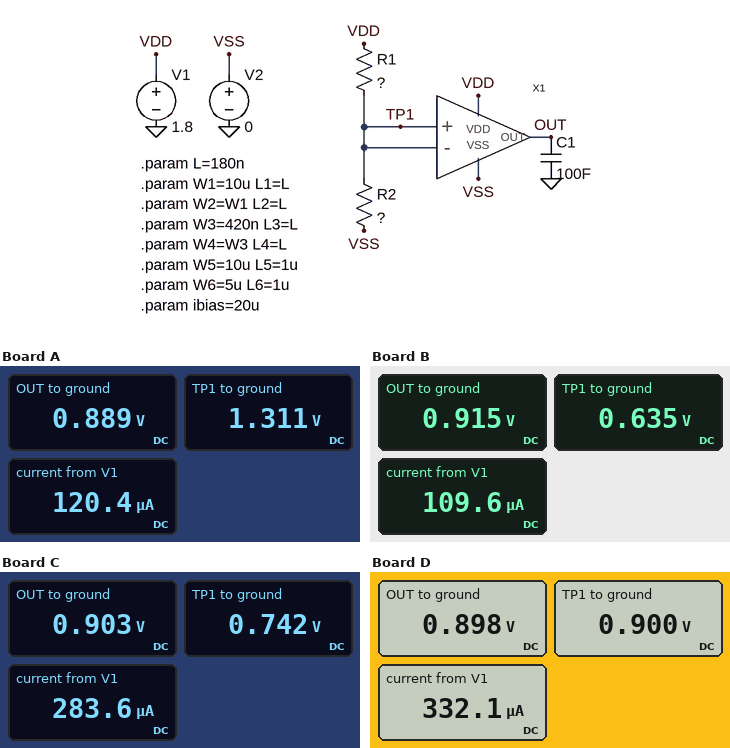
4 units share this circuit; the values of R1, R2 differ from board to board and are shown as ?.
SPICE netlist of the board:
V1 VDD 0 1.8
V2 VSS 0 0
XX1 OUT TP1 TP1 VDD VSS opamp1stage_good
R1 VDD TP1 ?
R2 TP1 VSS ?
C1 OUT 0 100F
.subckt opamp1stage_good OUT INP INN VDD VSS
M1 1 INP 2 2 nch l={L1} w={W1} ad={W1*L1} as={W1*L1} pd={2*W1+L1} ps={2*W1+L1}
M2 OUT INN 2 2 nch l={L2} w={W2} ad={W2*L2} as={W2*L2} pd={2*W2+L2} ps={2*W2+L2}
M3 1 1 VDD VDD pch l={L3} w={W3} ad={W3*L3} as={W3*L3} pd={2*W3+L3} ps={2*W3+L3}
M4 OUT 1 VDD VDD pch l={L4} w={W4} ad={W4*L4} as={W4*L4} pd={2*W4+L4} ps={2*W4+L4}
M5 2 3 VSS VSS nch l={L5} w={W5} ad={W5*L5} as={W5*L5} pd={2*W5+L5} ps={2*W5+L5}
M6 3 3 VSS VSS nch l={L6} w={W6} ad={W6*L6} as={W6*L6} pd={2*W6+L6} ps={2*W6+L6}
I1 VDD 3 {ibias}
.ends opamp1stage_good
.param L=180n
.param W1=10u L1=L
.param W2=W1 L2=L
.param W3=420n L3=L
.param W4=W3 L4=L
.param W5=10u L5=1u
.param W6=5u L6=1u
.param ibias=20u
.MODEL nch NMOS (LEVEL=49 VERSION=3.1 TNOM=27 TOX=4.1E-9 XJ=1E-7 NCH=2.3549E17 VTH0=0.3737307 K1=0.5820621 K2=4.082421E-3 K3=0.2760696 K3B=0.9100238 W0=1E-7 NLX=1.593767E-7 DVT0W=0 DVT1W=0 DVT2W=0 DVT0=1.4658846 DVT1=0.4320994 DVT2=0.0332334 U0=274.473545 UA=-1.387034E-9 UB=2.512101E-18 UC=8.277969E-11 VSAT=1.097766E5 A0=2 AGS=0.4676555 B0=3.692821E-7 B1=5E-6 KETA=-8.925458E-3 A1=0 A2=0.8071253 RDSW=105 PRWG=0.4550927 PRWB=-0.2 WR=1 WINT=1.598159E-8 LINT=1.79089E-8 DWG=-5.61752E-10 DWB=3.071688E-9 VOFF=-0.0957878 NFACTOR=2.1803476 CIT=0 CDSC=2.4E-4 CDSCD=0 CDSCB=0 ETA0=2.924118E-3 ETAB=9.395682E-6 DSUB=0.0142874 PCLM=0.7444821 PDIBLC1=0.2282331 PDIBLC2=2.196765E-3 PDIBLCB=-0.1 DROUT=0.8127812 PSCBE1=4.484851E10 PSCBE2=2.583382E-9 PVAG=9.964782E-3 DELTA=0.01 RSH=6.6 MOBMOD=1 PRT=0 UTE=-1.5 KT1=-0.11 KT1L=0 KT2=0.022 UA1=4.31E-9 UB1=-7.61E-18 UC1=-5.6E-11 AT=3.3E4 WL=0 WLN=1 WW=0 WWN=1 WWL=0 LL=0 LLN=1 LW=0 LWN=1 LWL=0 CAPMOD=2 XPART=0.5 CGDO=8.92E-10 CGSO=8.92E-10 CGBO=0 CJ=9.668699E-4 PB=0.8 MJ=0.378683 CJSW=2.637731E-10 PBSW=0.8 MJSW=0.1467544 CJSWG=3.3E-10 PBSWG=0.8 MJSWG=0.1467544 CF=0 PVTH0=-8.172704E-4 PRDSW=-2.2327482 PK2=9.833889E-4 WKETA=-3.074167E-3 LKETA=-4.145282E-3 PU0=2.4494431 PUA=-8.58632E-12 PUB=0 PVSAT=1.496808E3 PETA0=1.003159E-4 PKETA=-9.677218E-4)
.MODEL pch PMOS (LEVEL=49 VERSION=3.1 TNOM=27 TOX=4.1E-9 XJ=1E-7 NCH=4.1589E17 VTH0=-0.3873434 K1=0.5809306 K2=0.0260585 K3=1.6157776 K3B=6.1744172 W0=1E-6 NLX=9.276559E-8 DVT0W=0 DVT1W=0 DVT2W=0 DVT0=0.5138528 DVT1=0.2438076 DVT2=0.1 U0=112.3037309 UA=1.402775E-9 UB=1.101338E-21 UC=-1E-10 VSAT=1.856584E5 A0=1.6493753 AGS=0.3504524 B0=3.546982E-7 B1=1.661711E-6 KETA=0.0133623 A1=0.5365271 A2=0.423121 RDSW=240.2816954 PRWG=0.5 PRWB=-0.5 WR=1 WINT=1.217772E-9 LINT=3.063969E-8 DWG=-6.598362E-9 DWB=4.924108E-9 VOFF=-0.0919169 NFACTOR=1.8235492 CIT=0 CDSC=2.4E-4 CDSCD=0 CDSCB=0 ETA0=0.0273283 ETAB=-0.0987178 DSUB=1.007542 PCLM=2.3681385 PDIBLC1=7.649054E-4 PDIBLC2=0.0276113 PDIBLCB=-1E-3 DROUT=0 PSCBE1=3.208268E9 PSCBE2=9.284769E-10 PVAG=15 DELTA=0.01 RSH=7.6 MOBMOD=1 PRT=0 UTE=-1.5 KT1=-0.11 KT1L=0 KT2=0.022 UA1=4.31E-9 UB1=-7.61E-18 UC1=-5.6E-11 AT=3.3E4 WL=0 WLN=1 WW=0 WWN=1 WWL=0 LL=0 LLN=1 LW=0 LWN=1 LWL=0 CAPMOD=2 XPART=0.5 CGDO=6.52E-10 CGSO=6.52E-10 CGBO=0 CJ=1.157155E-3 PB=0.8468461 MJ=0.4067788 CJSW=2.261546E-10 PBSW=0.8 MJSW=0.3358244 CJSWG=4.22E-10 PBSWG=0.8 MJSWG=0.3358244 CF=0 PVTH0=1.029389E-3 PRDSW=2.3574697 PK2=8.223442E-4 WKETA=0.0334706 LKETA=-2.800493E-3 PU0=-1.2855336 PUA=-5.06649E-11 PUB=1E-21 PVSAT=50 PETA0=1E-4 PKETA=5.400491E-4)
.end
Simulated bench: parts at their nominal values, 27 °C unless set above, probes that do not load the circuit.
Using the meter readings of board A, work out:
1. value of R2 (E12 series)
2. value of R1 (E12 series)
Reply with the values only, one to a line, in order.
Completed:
22 kΩ
8.2 kΩ
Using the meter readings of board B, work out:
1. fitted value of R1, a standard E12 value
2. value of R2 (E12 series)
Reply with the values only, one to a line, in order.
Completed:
22 kΩ
12 kΩ
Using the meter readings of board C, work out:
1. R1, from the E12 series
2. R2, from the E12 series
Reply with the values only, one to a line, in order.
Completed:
4.7 kΩ
3.3 kΩ
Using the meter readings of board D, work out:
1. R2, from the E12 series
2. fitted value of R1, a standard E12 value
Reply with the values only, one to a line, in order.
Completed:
3.3 kΩ
3.3 kΩ
